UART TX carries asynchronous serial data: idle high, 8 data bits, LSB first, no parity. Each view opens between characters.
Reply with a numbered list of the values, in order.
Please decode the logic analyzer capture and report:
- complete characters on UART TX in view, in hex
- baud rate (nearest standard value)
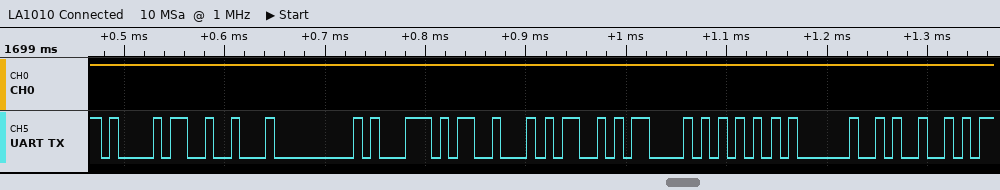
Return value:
1. A1, 12, 00, 71, 13, 4D, 43, 55, 20, 49
2. 115200 baud
